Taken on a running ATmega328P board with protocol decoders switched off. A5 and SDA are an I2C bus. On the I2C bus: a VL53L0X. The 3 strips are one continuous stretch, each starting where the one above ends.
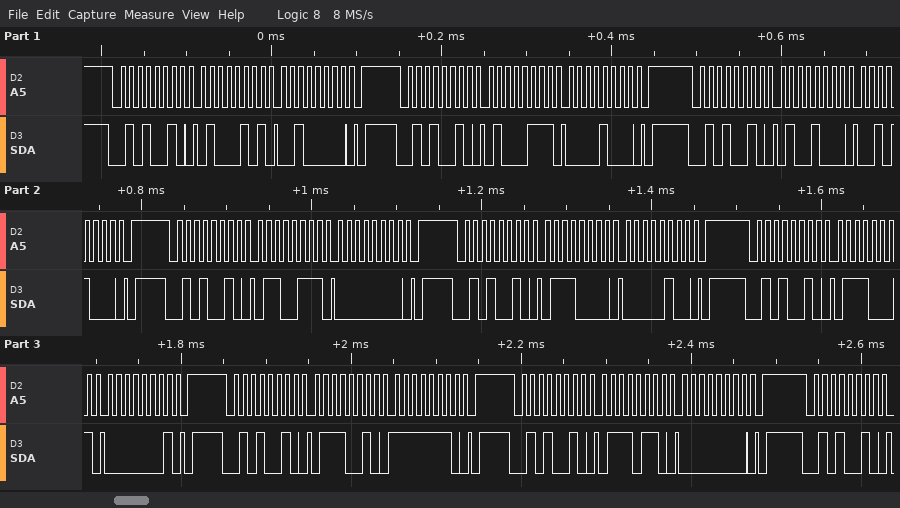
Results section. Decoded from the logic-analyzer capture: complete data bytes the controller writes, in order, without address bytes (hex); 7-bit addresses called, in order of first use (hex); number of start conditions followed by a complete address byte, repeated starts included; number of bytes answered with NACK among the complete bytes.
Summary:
45 20 47 08 48 28 67 00 70 04 71 01 72 FE 76 00
0x29
9
0
